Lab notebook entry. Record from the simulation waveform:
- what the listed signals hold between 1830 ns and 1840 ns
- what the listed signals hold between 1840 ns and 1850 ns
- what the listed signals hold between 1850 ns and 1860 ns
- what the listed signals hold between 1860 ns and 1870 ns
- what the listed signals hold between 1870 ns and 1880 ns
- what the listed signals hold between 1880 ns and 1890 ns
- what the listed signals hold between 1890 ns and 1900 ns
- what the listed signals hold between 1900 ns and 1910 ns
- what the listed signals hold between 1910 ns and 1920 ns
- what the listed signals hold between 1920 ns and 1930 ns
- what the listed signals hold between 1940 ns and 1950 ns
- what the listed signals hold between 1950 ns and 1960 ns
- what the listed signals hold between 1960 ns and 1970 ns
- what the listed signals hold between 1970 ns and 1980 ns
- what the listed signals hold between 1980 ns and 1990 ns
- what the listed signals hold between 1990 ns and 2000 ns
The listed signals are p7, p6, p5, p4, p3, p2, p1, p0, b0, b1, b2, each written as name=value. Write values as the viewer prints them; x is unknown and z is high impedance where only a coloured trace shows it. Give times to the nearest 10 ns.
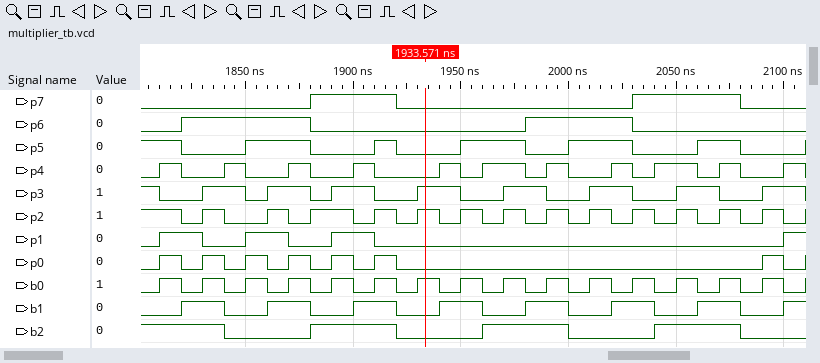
p7=0, p6=1, p5=0, p4=0, p3=1, p2=1, p1=0, p0=1, b0=1, b1=1, b2=1
p7=0, p6=1, p5=0, p4=1, p3=1, p2=0, p1=0, p0=0, b0=0, b1=0, b2=0
p7=0, p6=1, p5=1, p4=0, p3=0, p2=0, p1=1, p0=1, b0=1, b1=0, b2=0
p7=0, p6=1, p5=1, p4=0, p3=1, p2=1, p1=1, p0=0, b0=0, b1=1, b2=0
p7=0, p6=1, p5=1, p4=1, p3=1, p2=0, p1=0, p0=1, b0=1, b1=1, b2=0
p7=1, p6=0, p5=0, p4=0, p3=0, p2=1, p1=0, p0=0, b0=0, b1=0, b2=1
p7=1, p6=0, p5=0, p4=0, p3=1, p2=1, p1=1, p0=1, b0=1, b1=0, b2=1
p7=1, p6=0, p5=0, p4=1, p3=1, p2=0, p1=1, p0=0, b0=0, b1=1, b2=1
p7=1, p6=0, p5=1, p4=0, p3=0, p2=1, p1=0, p0=1, b0=1, b1=1, b2=1
p7=0, p6=0, p5=0, p4=0, p3=0, p2=0, p1=0, p0=0, b0=0, b1=0, b2=0
p7=0, p6=0, p5=0, p4=1, p3=1, p2=0, p1=0, p0=0, b0=0, b1=1, b2=0
p7=0, p6=0, p5=1, p4=0, p3=0, p2=1, p1=0, p0=0, b0=1, b1=1, b2=0
p7=0, p6=0, p5=1, p4=1, p3=0, p2=0, p1=0, p0=0, b0=0, b1=0, b2=1
p7=0, p6=0, p5=1, p4=1, p3=1, p2=1, p1=0, p0=0, b0=1, b1=0, b2=1
p7=0, p6=1, p5=0, p4=0, p3=1, p2=0, p1=0, p0=0, b0=0, b1=1, b2=1
p7=0, p6=1, p5=0, p4=1, p3=0, p2=1, p1=0, p0=0, b0=1, b1=1, b2=1
